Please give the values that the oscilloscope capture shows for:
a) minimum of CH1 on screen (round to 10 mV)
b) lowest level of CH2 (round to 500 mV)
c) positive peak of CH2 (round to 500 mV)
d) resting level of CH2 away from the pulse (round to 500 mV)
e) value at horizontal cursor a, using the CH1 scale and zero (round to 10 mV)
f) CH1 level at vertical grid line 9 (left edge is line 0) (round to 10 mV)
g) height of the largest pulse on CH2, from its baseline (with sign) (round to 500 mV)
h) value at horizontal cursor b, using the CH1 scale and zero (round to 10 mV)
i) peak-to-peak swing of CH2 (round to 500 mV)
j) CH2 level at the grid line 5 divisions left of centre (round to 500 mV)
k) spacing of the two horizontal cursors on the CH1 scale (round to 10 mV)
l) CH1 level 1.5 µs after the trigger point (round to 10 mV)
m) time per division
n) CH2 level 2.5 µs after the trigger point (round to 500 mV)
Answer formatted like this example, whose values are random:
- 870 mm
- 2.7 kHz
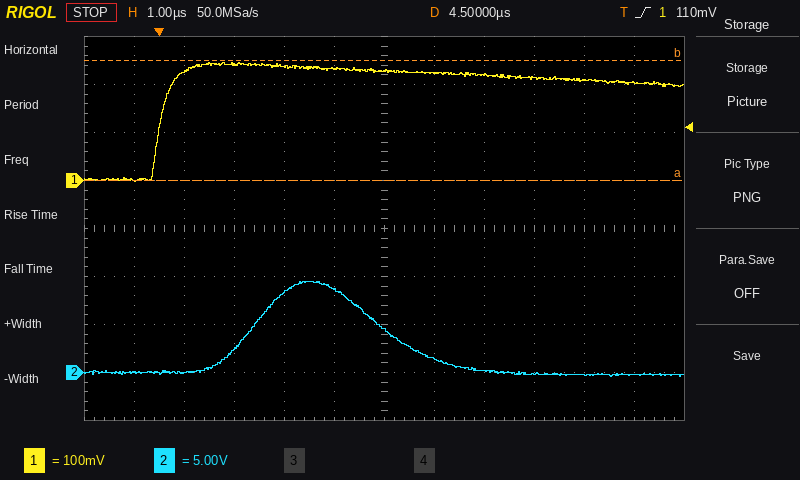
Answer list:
- 0 mV
- -500 mV
- 9.5 V
- 0.0 V
- 0 mV
- 210 mV
- +9.5 V
- 250 mV
- 10.0 V
- 0.0 V
- 250 mV
- 240 mV
- 1 µs
- 8.5 V
